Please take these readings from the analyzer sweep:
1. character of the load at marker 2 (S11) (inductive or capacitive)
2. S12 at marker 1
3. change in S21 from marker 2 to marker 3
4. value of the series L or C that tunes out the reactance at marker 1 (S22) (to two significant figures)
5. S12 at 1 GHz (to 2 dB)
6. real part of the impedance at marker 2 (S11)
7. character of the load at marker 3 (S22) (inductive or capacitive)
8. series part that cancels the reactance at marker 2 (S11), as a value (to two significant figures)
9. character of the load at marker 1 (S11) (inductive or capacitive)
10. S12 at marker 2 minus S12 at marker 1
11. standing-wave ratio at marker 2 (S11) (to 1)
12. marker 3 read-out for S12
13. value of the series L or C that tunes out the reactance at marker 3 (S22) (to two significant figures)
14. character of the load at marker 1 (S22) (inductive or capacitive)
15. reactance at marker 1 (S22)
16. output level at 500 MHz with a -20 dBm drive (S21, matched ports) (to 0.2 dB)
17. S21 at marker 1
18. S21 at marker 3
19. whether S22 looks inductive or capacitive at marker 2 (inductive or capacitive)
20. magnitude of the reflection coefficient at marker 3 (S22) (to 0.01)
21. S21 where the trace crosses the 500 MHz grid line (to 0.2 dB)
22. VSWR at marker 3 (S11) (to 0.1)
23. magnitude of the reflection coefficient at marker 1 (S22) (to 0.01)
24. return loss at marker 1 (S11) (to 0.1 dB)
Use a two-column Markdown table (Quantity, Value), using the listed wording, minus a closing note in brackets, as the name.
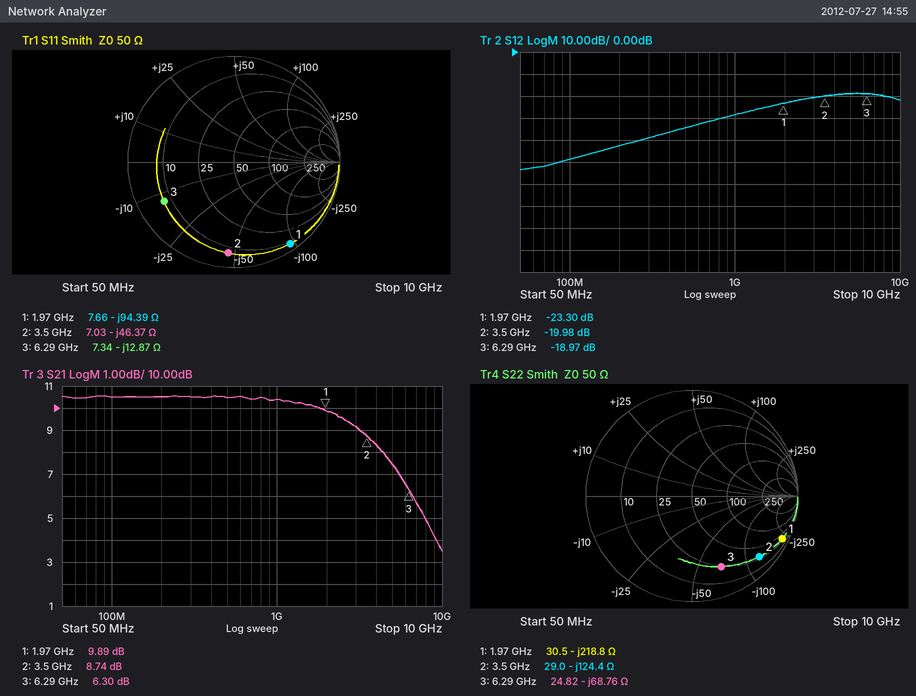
| Quantity | Value |
|---|---|
| character of the load at marker 2 (S11) | capacitive |
| S12 at marker 1 | -23.30 dB |
| change in S21 from marker 2 to marker 3 | -2.44 dB |
| value of the series L or C that tunes out the reactance at marker 1 (S22) | 18 nH |
| S12 at 1 GHz | -28 dB |
| real part of the impedance at marker 2 | 7.03 Ω |
| character of the load at marker 3 (S22) | capacitive |
| series part that cancels the reactance at marker 2 (S11), as a value | 2.1 nH |
| character of the load at marker 1 (S11) | capacitive |
| S12 at marker 2 minus S12 at marker 1 | 3.32 dB |
| standing-wave ratio at marker 2 (S11) | 13 |
| marker 3 read-out for S12 | -18.97 dB |
| value of the series L or C that tunes out the reactance at marker 3 (S22) | 1.7 nH |
| character of the load at marker 1 (S22) | capacitive |
| reactance at marker 1 | -218.8 Ω |
| output level at 500 MHz with a -20 dBm drive (S21, matched ports) | -9.6 dBm |
| S21 at marker 1 | 9.89 dB |
| S21 at marker 3 | 6.30 dB |
| whether S22 looks inductive or capacitive at marker 2 | capacitive |
| magnitude of the reflection coefficient at marker 3 (S22) | 0.72 |
| S21 where the trace crosses the 500 MHz grid line | 10.4 dB |
| VSWR at marker 3 (S11) | 7.3 |
| magnitude of the reflection coefficient at marker 1 (S22) | 0.94 |
| return loss at marker 1 (S11) | 0.6 dB |
